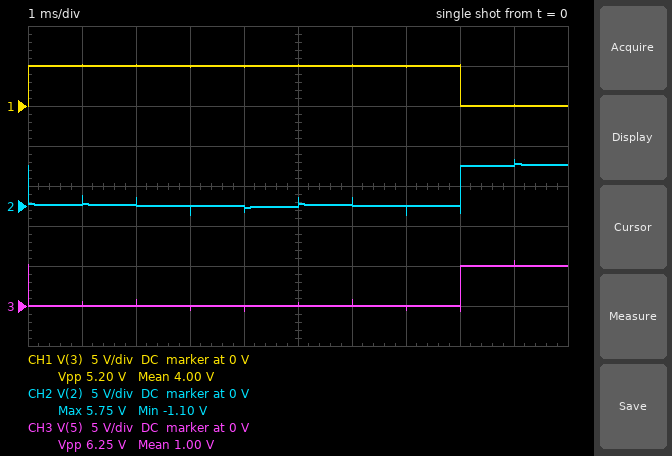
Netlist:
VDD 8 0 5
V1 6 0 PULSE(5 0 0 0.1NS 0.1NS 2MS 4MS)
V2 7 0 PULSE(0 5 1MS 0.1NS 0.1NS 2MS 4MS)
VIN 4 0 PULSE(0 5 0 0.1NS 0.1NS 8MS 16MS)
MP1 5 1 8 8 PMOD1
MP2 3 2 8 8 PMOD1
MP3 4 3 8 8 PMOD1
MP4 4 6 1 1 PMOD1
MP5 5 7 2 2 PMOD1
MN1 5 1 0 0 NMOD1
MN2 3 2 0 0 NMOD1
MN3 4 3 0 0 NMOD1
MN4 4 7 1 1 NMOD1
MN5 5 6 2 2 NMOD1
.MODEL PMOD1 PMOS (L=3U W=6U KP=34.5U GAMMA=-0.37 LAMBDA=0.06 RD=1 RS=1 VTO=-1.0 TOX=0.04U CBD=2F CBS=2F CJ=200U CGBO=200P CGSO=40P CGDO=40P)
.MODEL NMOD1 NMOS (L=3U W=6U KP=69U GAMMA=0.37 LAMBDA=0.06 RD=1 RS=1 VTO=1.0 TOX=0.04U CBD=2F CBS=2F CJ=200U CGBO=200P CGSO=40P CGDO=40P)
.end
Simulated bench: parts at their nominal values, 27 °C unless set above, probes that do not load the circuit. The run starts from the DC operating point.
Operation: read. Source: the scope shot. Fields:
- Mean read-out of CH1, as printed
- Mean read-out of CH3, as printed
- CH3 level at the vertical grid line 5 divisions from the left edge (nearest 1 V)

4.00 V
1.00 V
0 V
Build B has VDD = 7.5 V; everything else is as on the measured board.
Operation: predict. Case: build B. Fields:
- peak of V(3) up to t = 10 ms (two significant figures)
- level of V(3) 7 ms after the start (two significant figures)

7.6 V
7.5 V
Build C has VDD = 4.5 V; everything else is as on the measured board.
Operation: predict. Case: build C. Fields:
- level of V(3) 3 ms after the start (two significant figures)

4.5 V
